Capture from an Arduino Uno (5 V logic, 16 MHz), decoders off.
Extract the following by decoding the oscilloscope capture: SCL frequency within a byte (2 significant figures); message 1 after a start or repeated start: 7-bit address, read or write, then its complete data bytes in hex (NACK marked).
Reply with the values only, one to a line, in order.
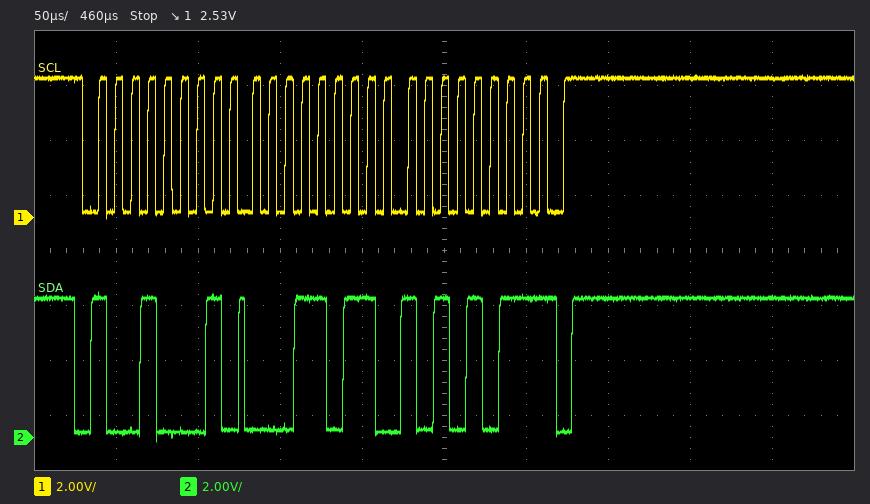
100 kHz
0x48 read: 1B AB NACK
